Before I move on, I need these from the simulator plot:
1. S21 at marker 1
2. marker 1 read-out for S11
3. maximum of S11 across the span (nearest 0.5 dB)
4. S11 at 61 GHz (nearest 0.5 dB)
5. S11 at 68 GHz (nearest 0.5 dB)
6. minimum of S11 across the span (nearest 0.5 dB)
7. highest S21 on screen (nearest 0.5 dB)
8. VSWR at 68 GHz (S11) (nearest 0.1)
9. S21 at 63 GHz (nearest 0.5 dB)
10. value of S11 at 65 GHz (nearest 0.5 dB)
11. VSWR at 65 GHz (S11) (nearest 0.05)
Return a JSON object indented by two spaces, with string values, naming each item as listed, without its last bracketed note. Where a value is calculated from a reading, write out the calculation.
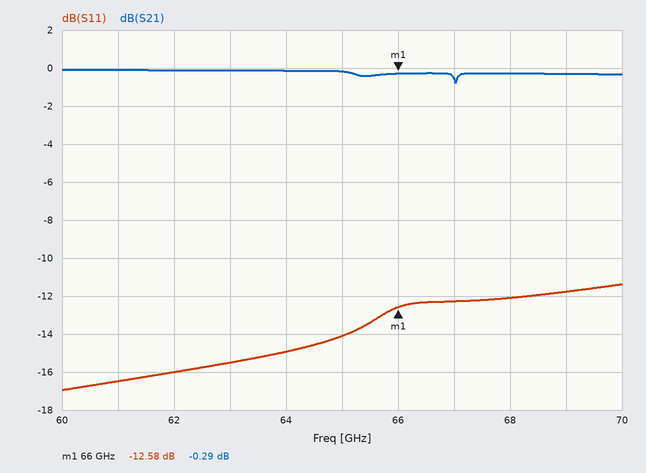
{
  "S21 at marker 1": "-0.29 dB",
  "marker 1 read-out for S11": "-12.58 dB",
  "maximum of S11 across the span": "-11.5 dB",
  "S11 at 61 GHz": "-16.5 dB",
  "S11 at 68 GHz": "-12.0 dB",
  "minimum of S11 across the span": "-17.0 dB",
  "highest S21 on screen": "0.0 dB",
  "VSWR at 68 GHz (S11)": "|Γ| = 10^(-12/20) = 0.2512; VSWR = (1 + 0.2512)/(1 − 0.2512) ≈ 1.7",
  "S21 at 63 GHz": "0.0 dB",
  "value of S11 at 65 GHz": "-14.0 dB",
  "VSWR at 65 GHz (S11)": "|Γ| = 10^(-14/20) = 0.1995; VSWR = (1 + 0.1995)/(1 − 0.1995) ≈ 1.50"
}
